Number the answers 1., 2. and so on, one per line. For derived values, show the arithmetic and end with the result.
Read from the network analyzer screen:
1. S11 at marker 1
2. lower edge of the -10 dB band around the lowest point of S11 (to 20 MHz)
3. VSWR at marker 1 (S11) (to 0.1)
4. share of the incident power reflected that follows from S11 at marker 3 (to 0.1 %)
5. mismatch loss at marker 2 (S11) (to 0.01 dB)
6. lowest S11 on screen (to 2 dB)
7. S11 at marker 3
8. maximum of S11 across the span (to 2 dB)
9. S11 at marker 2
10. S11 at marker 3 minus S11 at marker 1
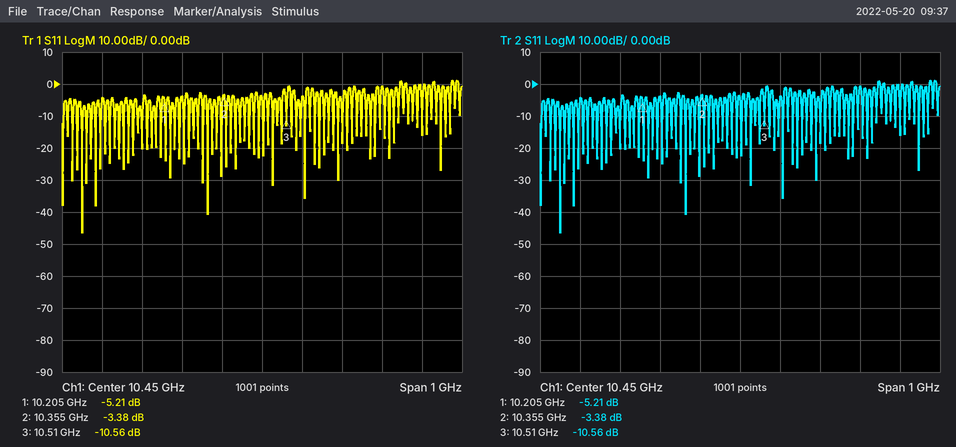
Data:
1. -5.21 dB
2. 10.00 GHz
3. (1 + 0.5489)/(1 − 0.5489) ≈ 3.4
4. 10^(-10.56/10) ≈ 8.8 %
5. −10 log10(1 − 10^(-3.38/10)) ≈ 2.67 dB
6. -46 dB
7. -10.56 dB
8. 2 dB
9. -3.38 dB
10. -10.56 − (-5.21) = -5.35 dB
